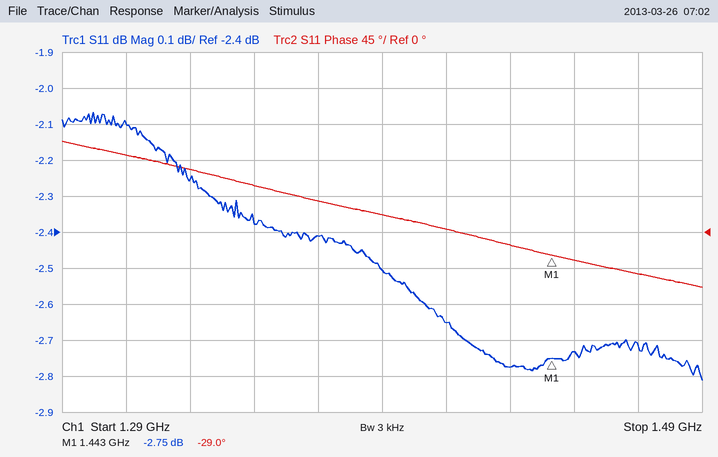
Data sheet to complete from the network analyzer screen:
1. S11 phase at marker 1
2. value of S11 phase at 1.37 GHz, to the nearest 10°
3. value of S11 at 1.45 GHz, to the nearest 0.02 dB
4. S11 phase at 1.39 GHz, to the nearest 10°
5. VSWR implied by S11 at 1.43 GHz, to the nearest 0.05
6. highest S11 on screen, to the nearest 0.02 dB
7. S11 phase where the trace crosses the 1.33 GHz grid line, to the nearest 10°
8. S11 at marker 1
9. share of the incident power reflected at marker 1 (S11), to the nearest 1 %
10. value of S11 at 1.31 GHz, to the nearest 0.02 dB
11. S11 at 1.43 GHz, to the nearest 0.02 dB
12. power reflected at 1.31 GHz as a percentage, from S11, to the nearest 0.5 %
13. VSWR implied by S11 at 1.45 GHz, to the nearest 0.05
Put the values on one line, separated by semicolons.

-29.0°; 40°; -2.74 dB; 20°; 6.30; -2.06 dB; 80°; -2.75 dB; 53 %; -2.10 dB; -2.78 dB; 61.5 %; 6.40
